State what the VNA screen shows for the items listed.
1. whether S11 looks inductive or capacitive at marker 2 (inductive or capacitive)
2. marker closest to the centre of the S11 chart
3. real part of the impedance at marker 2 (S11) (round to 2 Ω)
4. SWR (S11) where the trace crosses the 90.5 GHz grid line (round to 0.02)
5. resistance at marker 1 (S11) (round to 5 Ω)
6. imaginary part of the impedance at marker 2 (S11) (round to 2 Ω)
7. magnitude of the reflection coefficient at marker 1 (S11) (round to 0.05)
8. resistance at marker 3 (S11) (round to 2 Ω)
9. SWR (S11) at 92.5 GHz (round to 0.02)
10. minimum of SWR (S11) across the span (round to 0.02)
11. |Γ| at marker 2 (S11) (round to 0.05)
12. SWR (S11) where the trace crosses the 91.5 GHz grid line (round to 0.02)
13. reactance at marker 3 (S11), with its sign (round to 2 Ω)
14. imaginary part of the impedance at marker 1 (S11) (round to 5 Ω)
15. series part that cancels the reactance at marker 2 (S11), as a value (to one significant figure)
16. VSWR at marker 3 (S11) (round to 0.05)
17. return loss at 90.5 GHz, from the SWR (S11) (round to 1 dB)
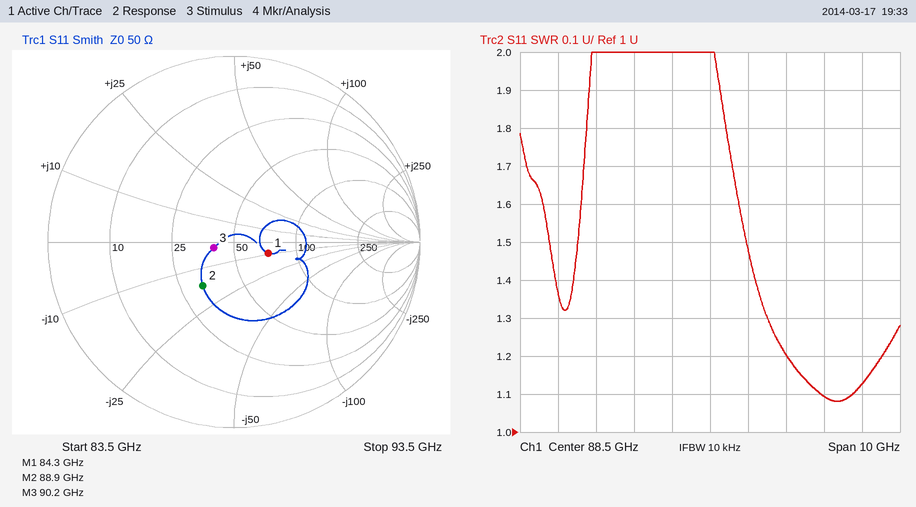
capacitive
marker 3
32 Ω
1.20
70 Ω
-16 Ω
0.20
40 Ω
1.12
1.08
0.30
1.10
-2 Ω
-10 Ω
30 pH
1.25
21 dB
